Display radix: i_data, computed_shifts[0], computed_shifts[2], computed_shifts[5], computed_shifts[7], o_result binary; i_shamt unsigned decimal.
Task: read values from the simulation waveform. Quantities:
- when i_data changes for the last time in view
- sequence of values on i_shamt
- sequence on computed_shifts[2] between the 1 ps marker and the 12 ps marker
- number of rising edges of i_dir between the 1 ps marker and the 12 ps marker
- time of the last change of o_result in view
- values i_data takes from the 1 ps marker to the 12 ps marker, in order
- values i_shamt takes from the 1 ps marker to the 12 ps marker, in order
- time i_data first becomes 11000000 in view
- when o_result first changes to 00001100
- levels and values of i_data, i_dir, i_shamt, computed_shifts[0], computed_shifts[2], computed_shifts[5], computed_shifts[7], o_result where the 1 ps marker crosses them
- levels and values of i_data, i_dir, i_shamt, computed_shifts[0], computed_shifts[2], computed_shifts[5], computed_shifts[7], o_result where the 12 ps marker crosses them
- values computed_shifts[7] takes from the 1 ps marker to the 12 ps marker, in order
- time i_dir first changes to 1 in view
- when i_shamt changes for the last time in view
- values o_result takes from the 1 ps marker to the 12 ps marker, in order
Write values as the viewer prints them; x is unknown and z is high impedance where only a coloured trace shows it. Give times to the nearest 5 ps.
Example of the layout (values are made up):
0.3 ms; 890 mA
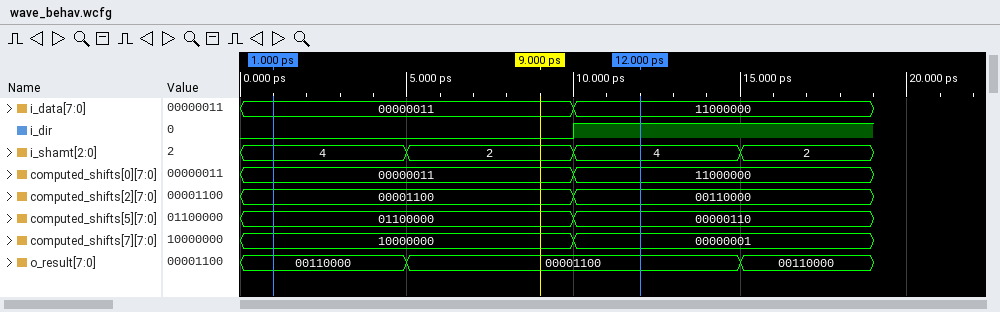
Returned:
10 ps; 4, 2, 4, 2; 00001100, 00110000; 1; 15 ps; 00000011, 11000000; 4, 2, 4; 10 ps; 5 ps; i_data=00000011, i_dir=0, i_shamt=4, computed_shifts[0]=00000011, computed_shifts[2]=00001100, computed_shifts[5]=01100000, computed_shifts[7]=10000000, o_result=00110000; i_data=11000000, i_dir=1, i_shamt=4, computed_shifts[0]=11000000, computed_shifts[2]=00110000, computed_shifts[5]=00000110, computed_shifts[7]=00000001, o_result=00001100; 10000000, 00000001; 10 ps; 15 ps; 00110000, 00001100
